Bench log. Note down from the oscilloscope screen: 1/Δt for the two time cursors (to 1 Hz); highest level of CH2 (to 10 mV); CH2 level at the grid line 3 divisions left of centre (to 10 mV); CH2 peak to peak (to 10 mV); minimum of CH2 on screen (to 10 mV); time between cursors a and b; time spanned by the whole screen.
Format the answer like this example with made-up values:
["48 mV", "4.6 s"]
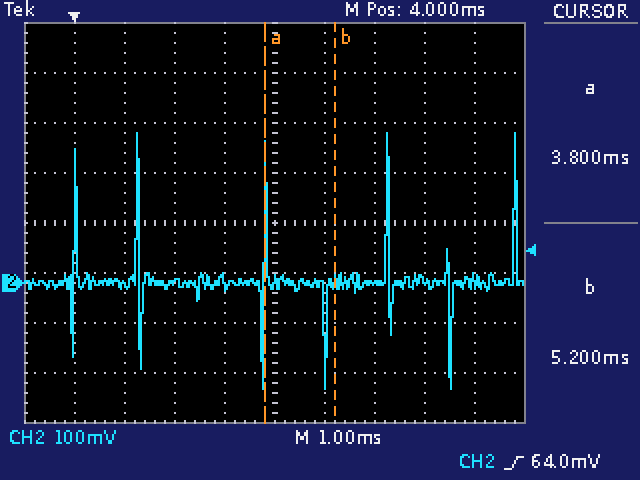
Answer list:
["714 Hz", "300 mV", "0 mV", "510 mV", "-210 mV", "1.4 ms", "10 ms"]
